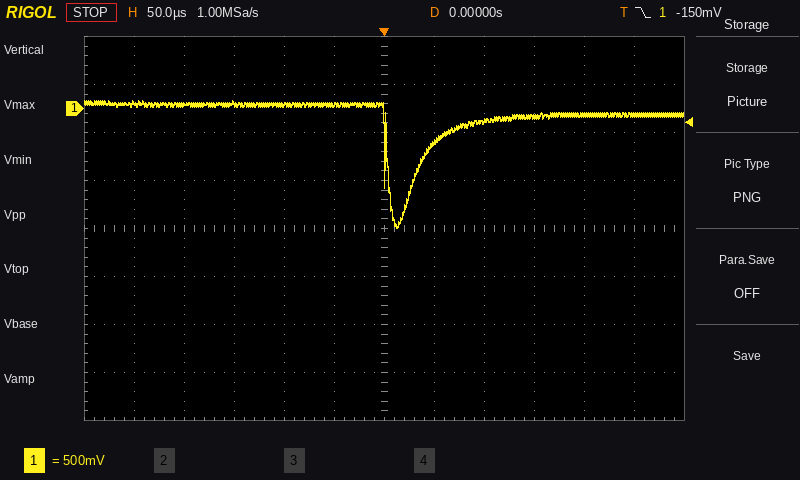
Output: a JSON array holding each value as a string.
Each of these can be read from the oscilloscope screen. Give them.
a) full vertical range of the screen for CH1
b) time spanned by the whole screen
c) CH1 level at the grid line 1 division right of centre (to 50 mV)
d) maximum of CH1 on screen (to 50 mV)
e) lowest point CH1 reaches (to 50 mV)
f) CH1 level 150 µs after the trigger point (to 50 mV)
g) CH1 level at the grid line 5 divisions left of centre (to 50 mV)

["4 V", "600 µs", "-350 mV", "100 mV", "-1.25 V", "-100 mV", "50 mV"]
